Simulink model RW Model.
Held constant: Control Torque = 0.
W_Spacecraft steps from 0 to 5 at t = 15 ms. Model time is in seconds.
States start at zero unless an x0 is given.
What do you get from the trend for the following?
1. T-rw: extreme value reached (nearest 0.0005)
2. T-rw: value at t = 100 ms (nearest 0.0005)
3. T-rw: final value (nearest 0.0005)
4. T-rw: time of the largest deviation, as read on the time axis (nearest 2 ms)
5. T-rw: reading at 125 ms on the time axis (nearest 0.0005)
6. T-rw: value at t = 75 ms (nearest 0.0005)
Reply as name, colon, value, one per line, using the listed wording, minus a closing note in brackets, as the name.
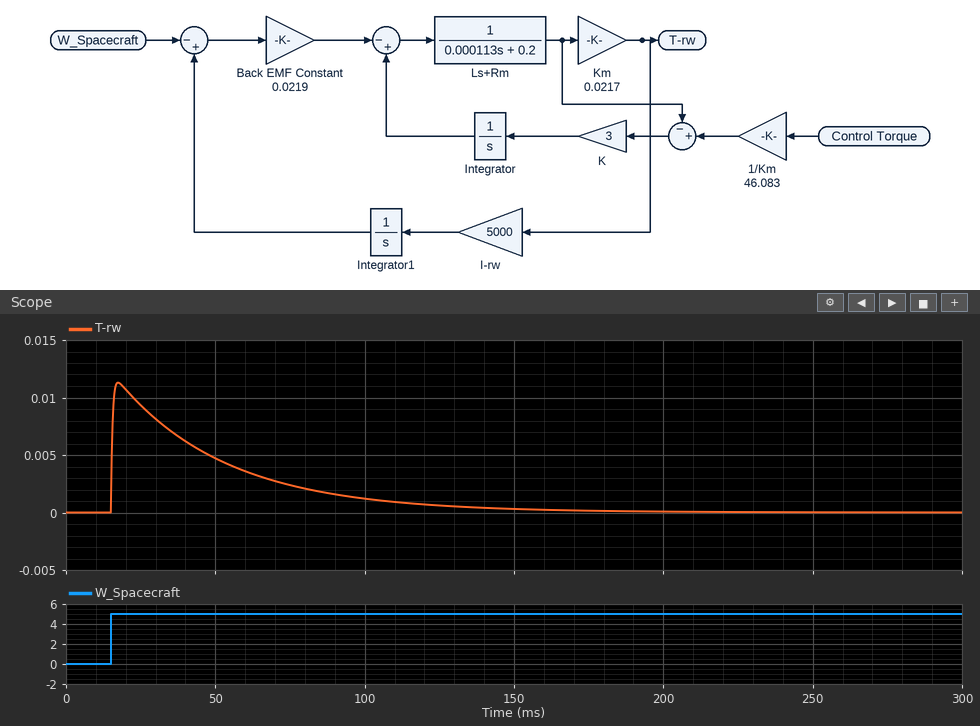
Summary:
T-rw: extreme value reached: 0.0115
T-rw: value at t = 100 ms: 0.0010
T-rw: final value: 0.0000
T-rw: time of the largest deviation, as read on the time axis: 18 ms
T-rw: reading at 125 ms on the time axis: 0.0005
T-rw: value at t = 75 ms: 0.0025
